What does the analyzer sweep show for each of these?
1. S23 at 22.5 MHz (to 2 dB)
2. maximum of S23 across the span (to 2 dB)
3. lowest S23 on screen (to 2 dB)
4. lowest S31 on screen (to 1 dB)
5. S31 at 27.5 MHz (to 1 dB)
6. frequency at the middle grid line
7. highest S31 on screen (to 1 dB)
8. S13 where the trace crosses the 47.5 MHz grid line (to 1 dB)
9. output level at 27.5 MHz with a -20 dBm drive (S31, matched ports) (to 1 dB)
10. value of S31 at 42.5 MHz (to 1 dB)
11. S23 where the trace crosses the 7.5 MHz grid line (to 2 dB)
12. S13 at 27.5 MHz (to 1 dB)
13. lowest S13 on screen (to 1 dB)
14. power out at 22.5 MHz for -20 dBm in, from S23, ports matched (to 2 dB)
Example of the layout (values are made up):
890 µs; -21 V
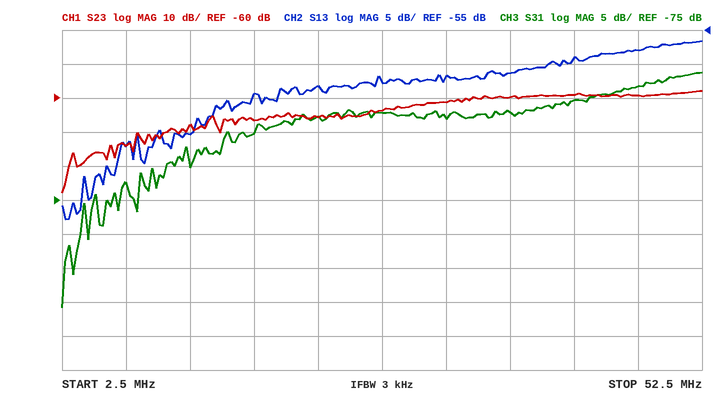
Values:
-66 dB; -58 dB; -88 dB; -91 dB; -62 dB; 27.5 MHz; -56 dB; -58 dB; -82 dBm; -60 dB; -74 dB; -63 dB; -83 dB; -86 dBm
